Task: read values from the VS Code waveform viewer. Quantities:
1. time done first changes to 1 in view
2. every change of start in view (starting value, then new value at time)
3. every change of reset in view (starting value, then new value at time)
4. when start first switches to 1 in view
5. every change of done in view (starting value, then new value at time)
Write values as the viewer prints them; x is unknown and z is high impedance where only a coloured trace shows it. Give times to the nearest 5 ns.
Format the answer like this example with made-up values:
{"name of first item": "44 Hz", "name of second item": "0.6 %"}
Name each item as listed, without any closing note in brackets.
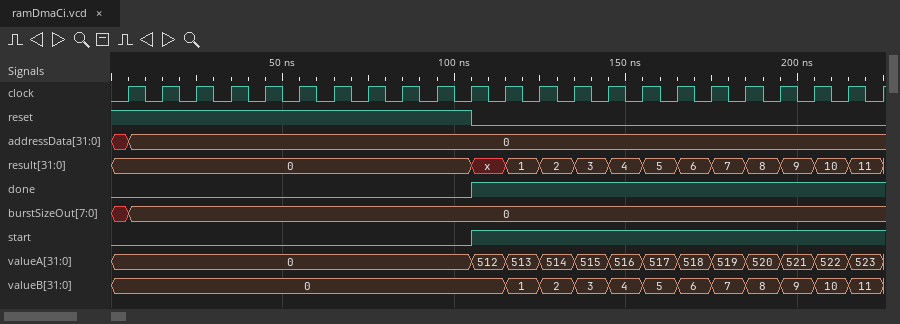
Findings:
{"time done first changes to 1 in view": "105 ns", "every change of start in view": "0, 1 at 105 ns", "every change of reset in view": "1, 0 at 105 ns", "when start first switches to 1 in view": "105 ns", "every change of done in view": "0, 1 at 105 ns"}
